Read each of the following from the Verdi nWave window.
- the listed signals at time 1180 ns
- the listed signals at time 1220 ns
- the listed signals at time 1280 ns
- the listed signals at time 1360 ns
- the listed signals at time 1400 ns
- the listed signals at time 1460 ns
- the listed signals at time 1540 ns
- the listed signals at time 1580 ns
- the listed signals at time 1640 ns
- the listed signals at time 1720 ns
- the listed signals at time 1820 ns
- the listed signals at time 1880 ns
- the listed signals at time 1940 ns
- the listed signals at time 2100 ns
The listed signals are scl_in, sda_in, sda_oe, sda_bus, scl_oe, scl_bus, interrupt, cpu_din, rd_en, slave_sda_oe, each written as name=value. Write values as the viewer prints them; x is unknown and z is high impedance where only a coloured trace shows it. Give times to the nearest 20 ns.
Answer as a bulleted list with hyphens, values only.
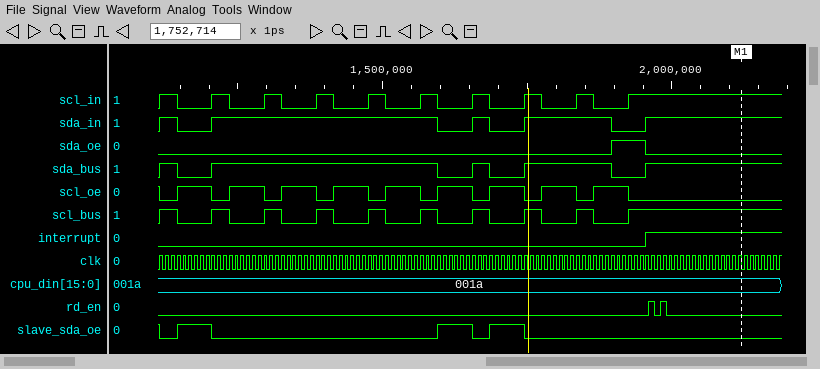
- scl_in=0, sda_in=0, sda_oe=0, sda_bus=0, scl_oe=1, scl_bus=0, interrupt=0, cpu_din=001a, rd_en=0, slave_sda_oe=1
- scl_in=1, sda_in=1, sda_oe=0, sda_bus=1, scl_oe=0, scl_bus=1, interrupt=0, cpu_din=001a, rd_en=0, slave_sda_oe=0
- scl_in=0, sda_in=1, sda_oe=0, sda_bus=1, scl_oe=1, scl_bus=0, interrupt=0, cpu_din=001a, rd_en=0, slave_sda_oe=0
- scl_in=0, sda_in=1, sda_oe=0, sda_bus=1, scl_oe=1, scl_bus=0, interrupt=0, cpu_din=001a, rd_en=0, slave_sda_oe=0
- scl_in=1, sda_in=1, sda_oe=0, sda_bus=1, scl_oe=0, scl_bus=1, interrupt=0, cpu_din=001a, rd_en=0, slave_sda_oe=0
- scl_in=0, sda_in=1, sda_oe=0, sda_bus=1, scl_oe=1, scl_bus=0, interrupt=0, cpu_din=001a, rd_en=0, slave_sda_oe=0
- scl_in=0, sda_in=1, sda_oe=0, sda_bus=1, scl_oe=1, scl_bus=0, interrupt=0, cpu_din=001a, rd_en=0, slave_sda_oe=0
- scl_in=1, sda_in=1, sda_oe=0, sda_bus=1, scl_oe=0, scl_bus=1, interrupt=0, cpu_din=001a, rd_en=0, slave_sda_oe=0
- scl_in=0, sda_in=0, sda_oe=0, sda_bus=0, scl_oe=1, scl_bus=0, interrupt=0, cpu_din=001a, rd_en=0, slave_sda_oe=1
- scl_in=0, sda_in=0, sda_oe=0, sda_bus=0, scl_oe=1, scl_bus=0, interrupt=0, cpu_din=001a, rd_en=0, slave_sda_oe=1
- scl_in=0, sda_in=1, sda_oe=0, sda_bus=1, scl_oe=1, scl_bus=0, interrupt=0, cpu_din=001a, rd_en=0, slave_sda_oe=0
- scl_in=0, sda_in=1, sda_oe=0, sda_bus=1, scl_oe=1, scl_bus=0, interrupt=0, cpu_din=001a, rd_en=0, slave_sda_oe=0
- scl_in=1, sda_in=0, sda_oe=1, sda_bus=0, scl_oe=0, scl_bus=1, interrupt=0, cpu_din=001a, rd_en=0, slave_sda_oe=0
- scl_in=1, sda_in=1, sda_oe=0, sda_bus=1, scl_oe=0, scl_bus=1, interrupt=1, cpu_din=001a, rd_en=0, slave_sda_oe=0
